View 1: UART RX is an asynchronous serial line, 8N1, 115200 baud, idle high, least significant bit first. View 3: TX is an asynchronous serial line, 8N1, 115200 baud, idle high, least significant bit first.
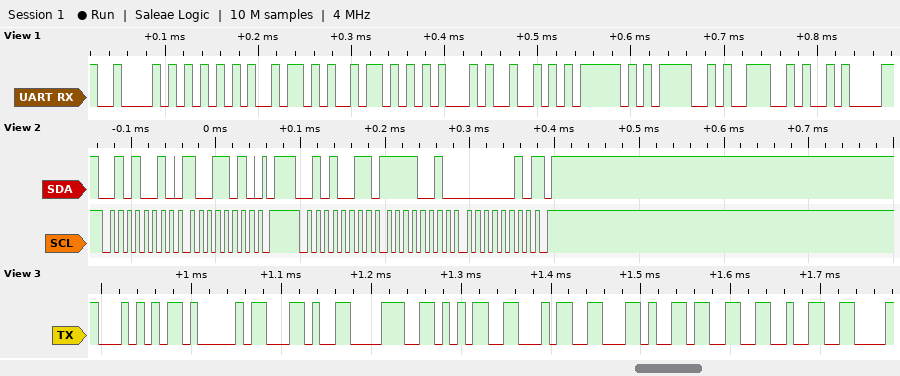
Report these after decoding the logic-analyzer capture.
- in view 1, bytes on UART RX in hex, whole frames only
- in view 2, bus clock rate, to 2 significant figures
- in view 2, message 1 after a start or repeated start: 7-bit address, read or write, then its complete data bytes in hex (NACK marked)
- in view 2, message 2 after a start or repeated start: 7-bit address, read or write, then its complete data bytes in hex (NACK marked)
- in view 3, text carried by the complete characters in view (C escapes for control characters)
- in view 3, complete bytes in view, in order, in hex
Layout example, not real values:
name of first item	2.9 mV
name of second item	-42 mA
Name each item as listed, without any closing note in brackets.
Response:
in view 1, bytes on UART RX in hex, whole frames only	42 55 5A 5A 45 52 5F 4F 4E 0A
in view 2, bus clock rate, to 2 significant figures	100 kHz
in view 2, message 1 after a start or repeated start: 7-bit address, read or write, then its complete data bytes in hex	0x29 write: 9A
in view 2, message 2 after a start or repeated start: 7-bit address, read or write, then its complete data bytes in hex	0x29 read: F2 02 NACK
in view 3, text carried by the complete characters in view	"TA,854,32"
in view 3, complete bytes in view, in order, in hex	54 41 2C 38 35 34 2C 33 32
